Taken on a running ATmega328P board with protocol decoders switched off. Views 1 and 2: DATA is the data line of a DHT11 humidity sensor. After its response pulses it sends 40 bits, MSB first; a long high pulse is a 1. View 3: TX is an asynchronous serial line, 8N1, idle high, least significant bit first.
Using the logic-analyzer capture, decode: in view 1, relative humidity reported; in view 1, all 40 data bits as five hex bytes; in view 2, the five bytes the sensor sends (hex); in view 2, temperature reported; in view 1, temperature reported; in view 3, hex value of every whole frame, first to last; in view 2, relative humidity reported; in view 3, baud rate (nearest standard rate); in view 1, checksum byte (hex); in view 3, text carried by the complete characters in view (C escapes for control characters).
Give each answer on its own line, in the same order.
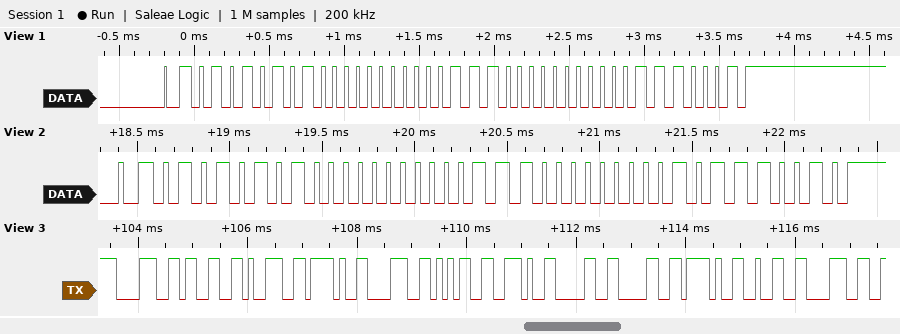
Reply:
85 %
55 00 1C 00 71
55 00 1C 01 72
28.1 °C
28.0 °C
0x38 0x33 0x39 0x2F 0x38 0x35 0x2E 0x30 0x30 0x2F 0x32 0x38
85 %
9600 baud
0x71
"839/85.00/28"
